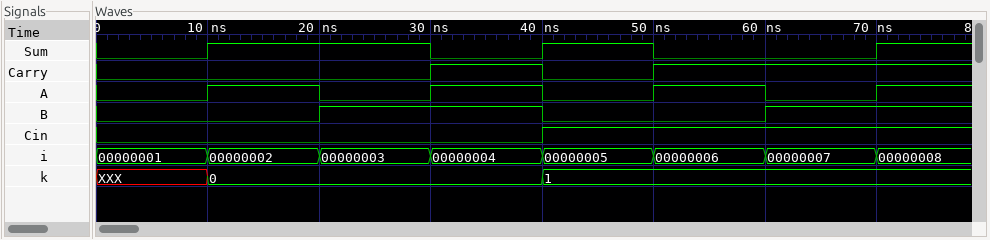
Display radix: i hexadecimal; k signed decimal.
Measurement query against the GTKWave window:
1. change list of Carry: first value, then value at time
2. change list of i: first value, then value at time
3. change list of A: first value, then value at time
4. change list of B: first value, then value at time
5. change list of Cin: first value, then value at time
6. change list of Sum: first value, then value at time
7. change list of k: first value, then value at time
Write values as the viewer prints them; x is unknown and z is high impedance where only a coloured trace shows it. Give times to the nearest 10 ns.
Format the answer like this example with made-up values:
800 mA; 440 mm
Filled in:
0, 1 at 30 ns, 0 at 40 ns, 1 at 50 ns; 00000001, 00000002 at 10 ns, 00000003 at 20 ns, 00000004 at 30 ns, 00000005 at 40 ns, 00000006 at 50 ns, 00000007 at 60 ns, 00000008 at 70 ns; 0, 1 at 10 ns, 0 at 20 ns, 1 at 30 ns, 0 at 40 ns, 1 at 50 ns, 0 at 60 ns, 1 at 70 ns; 0, 1 at 20 ns, 0 at 40 ns, 1 at 60 ns; 0, 1 at 40 ns; 0, 1 at 10 ns, 0 at 30 ns, 1 at 40 ns, 0 at 50 ns, 1 at 70 ns; XXX, 0 at 10 ns, 1 at 40 ns
